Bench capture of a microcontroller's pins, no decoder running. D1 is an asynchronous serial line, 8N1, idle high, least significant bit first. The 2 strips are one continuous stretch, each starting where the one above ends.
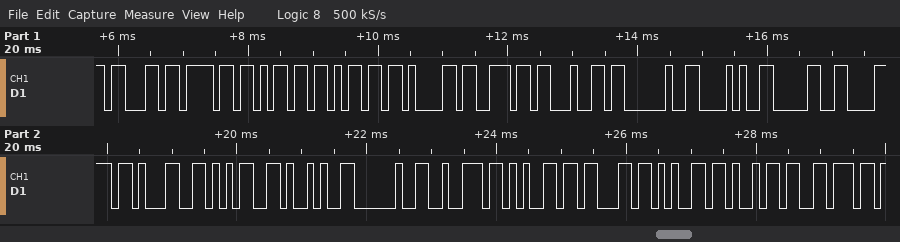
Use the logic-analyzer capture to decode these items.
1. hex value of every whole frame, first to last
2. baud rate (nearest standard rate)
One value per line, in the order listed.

63 6F 6D 6D 61 6E 64 20 28 30 78 31 35 29 20 72 65 63 65 69 76
9600 baud
